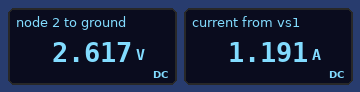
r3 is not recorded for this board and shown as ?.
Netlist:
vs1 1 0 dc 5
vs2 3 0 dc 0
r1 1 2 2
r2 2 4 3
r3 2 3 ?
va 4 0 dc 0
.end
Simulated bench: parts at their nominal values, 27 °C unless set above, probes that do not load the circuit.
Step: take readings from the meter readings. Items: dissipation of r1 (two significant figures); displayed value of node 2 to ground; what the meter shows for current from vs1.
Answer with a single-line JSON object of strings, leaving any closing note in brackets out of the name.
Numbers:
{"dissipation of r1": "2.8 W", "displayed value of node 2 to ground": "2.617 V", "what the meter shows for current from vs1": "1.191 A"}
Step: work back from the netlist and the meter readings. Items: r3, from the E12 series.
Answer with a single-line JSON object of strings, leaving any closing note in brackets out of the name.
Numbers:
{"r3, from the E12 series": "8.2 Ω"}
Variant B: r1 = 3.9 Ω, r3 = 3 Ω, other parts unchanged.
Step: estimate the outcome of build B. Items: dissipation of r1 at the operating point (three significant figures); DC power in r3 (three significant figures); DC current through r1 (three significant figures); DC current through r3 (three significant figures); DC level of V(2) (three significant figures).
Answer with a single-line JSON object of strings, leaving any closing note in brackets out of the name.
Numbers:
{"dissipation of r1 at the operating point": "3.34 W", "DC power in r3": "643 mW", "DC current through r1": "926 mA", "DC current through r3": "463 mA", "DC level of V(2)": "1.39 V"}
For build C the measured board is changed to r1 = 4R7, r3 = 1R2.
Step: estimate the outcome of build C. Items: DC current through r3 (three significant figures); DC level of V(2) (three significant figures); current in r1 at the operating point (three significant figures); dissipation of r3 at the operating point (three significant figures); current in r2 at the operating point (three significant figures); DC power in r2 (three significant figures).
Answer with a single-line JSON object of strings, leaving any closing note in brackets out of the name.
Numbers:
{"DC current through r3": "643 mA", "DC level of V(2)": "771 mV", "current in r1 at the operating point": "900 mA", "dissipation of r3 at the operating point": "496 mW", "current in r2 at the operating point": "257 mA", "DC power in r2": "198 mW"}
